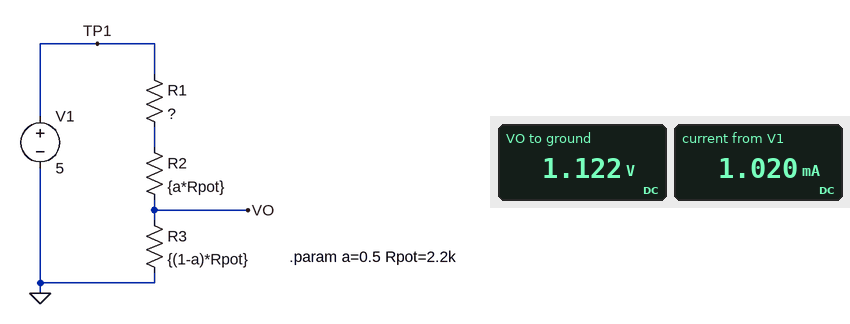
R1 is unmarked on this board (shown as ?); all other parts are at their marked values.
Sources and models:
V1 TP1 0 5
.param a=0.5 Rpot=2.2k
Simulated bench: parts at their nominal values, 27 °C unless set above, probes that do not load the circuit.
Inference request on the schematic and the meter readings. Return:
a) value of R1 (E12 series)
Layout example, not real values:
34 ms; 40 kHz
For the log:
2.7 kΩ
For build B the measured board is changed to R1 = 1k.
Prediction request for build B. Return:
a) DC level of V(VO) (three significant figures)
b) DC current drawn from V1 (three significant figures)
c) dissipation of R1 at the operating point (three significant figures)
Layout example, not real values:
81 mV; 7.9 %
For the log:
1.72 V; 1.56 mA; 2.44 mW
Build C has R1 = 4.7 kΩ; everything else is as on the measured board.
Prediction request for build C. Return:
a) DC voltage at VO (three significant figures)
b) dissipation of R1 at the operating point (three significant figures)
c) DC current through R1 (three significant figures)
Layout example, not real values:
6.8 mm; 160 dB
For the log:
797 mV; 2.47 mW; 725 µA
